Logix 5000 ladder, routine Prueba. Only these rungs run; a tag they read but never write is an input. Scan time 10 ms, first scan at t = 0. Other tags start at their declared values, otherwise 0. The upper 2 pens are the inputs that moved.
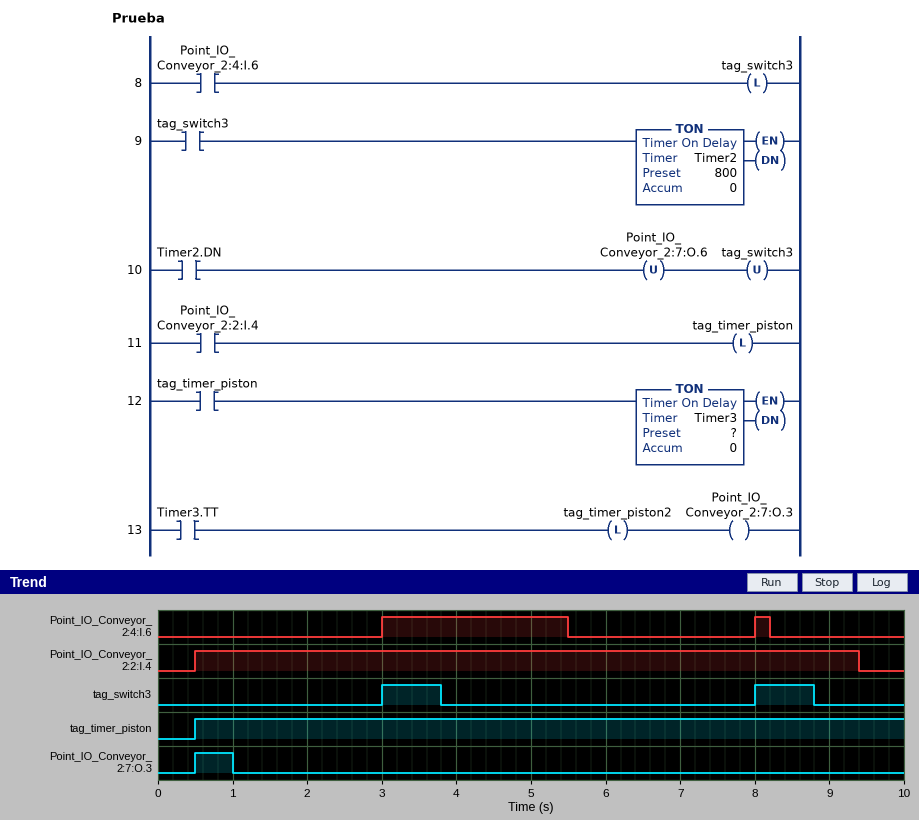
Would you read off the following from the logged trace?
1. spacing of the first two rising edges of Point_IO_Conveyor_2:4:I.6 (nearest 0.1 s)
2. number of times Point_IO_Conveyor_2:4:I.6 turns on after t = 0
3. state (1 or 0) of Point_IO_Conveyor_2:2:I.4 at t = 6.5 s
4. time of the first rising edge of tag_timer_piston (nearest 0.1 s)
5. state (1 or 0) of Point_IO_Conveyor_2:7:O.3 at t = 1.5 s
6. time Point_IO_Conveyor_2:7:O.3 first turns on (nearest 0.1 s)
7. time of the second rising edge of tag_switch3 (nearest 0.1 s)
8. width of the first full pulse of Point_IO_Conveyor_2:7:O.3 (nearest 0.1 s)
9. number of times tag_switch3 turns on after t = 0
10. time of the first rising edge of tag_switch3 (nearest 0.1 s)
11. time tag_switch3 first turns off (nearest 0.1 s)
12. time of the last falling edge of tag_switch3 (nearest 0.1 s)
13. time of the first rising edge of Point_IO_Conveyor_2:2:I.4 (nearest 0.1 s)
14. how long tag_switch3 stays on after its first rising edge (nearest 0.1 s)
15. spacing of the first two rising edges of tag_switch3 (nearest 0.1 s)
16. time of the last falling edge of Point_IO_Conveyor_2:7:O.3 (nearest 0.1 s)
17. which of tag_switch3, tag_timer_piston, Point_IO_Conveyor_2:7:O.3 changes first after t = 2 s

5.0 s
2
1
0.5 s
0
0.5 s
8.0 s
0.5 s
2
3.0 s
3.8 s
8.8 s
0.5 s
0.8 s
5.0 s
1.0 s
tag_switch3
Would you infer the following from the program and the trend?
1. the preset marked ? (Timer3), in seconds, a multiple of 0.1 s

0.5 s
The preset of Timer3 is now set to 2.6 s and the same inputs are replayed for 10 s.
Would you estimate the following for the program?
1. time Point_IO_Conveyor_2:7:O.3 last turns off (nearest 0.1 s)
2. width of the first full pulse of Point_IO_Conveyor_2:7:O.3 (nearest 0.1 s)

3.1 s
2.6 s
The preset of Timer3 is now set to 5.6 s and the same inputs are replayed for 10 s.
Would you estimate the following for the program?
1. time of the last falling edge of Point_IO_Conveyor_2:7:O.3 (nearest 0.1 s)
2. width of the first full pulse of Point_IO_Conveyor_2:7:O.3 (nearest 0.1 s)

6.1 s
5.6 s
